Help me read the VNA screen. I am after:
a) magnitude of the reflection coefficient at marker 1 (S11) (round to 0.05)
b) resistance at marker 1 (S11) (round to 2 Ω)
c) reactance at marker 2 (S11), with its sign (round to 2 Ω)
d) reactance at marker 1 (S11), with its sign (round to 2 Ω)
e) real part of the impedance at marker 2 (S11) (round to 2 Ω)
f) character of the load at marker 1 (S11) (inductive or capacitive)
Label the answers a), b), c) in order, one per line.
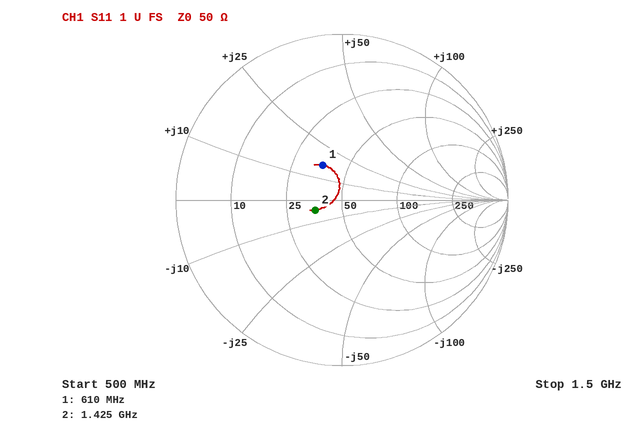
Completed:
a) 0.25
b) 36 Ω
c) -4 Ω
d) +16 Ω
e) 36 Ω
f) inductive
